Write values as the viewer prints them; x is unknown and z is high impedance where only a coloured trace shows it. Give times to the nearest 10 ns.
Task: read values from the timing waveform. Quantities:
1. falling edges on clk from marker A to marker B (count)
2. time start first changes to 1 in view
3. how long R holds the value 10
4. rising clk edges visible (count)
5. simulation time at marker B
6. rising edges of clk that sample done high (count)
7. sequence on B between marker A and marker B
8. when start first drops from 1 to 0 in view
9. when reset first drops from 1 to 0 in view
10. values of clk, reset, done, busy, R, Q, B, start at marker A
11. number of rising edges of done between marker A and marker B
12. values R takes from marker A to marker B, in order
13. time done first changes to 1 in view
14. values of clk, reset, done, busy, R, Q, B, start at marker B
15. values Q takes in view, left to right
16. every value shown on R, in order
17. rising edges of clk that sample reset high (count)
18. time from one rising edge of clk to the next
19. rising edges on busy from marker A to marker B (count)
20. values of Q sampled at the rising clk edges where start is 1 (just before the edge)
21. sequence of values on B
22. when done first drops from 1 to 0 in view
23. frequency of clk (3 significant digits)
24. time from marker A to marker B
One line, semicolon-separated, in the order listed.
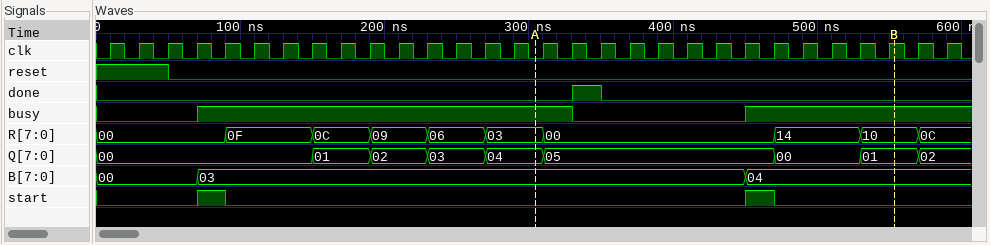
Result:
12; 70 ns; 40 ns; 30; 550 ns; 1; 03, 04; 90 ns; 50 ns; clk=0, reset=0, done=0, busy=1, R=03, Q=04, B=03, start=0; 1; 03, 00, 14, 10; 330 ns; clk=1, reset=0, done=0, busy=1, R=10, Q=01, B=04, start=0; 00, 01, 02, 03, 04, 05, 00, 01, 02; 00, 0F, 0C, 09, 06, 03, 00, 14, 10, 0C; 3; 20 ns; 1; 00, 05; 00, 03, 04; 350 ns; 50.0 MHz; 250 ns
